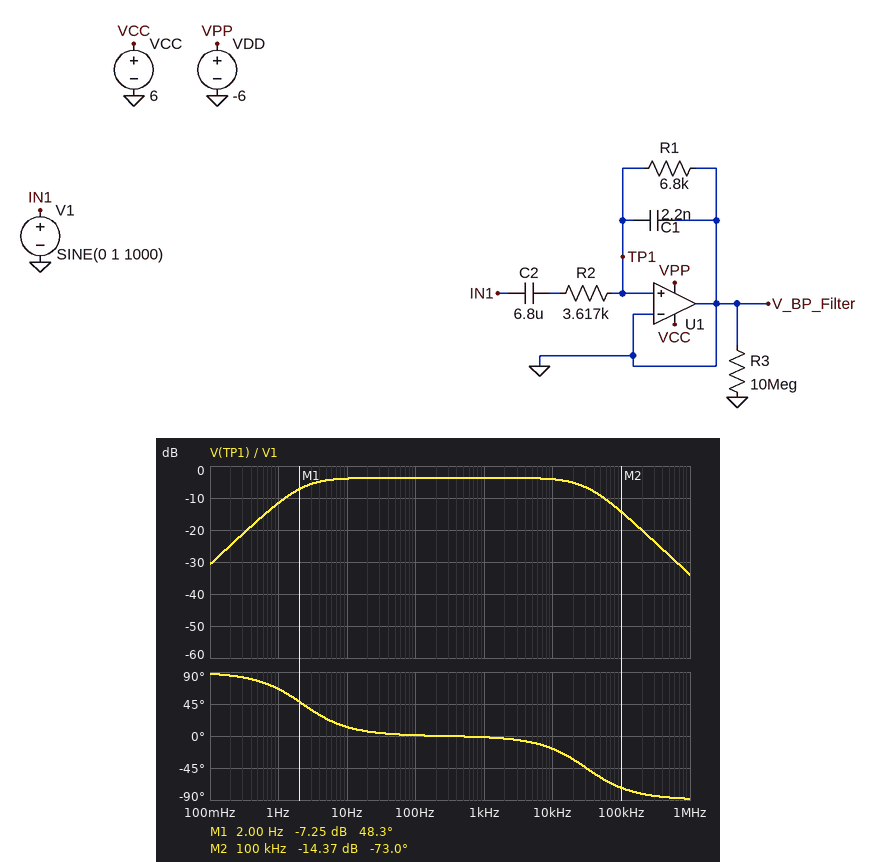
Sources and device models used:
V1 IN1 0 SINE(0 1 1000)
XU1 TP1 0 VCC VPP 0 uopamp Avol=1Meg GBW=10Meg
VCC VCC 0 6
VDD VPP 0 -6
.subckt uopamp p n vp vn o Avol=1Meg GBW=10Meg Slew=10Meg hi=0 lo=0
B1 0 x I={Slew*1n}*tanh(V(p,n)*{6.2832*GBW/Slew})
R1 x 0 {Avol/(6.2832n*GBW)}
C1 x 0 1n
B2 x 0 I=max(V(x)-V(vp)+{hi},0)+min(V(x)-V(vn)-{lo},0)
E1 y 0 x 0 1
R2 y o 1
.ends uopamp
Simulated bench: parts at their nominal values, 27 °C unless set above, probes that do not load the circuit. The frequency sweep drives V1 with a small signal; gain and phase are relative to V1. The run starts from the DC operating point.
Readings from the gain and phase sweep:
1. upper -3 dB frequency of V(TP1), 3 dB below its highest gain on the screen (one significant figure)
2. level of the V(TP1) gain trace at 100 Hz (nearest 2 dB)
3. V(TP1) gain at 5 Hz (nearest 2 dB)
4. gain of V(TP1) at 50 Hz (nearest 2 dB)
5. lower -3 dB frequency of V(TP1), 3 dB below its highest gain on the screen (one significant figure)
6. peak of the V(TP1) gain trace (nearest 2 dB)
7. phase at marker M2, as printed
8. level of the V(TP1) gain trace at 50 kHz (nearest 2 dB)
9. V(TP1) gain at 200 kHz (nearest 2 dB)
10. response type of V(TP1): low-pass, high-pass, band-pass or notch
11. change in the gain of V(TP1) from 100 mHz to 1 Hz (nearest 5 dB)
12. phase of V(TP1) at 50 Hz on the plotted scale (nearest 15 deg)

30 kHz
-4 dB
-4 dB
-4 dB
2 Hz
-4 dB
-73.0 deg
-10 dB
-20 dB
band-pass
20 dB
0 deg
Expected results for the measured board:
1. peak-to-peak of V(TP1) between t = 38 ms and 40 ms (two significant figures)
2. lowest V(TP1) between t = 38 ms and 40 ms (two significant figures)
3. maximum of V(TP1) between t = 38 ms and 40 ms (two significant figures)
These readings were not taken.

1.3 V
-650 mV
650 mV
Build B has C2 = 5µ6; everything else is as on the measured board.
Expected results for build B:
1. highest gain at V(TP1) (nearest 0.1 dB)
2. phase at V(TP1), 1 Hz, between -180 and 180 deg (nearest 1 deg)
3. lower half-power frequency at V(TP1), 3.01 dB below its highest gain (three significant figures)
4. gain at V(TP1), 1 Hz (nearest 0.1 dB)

-3.7 dB
70 deg
2.73 Hz
-13.0 dB
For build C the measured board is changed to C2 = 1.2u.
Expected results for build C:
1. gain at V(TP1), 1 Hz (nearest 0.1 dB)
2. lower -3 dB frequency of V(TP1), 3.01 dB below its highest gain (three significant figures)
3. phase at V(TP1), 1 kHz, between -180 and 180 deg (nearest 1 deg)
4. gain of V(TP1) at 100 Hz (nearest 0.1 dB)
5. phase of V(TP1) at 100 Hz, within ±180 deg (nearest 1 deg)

-25.8 dB
12.7 Hz
-1 deg
-3.8 dB
7 deg
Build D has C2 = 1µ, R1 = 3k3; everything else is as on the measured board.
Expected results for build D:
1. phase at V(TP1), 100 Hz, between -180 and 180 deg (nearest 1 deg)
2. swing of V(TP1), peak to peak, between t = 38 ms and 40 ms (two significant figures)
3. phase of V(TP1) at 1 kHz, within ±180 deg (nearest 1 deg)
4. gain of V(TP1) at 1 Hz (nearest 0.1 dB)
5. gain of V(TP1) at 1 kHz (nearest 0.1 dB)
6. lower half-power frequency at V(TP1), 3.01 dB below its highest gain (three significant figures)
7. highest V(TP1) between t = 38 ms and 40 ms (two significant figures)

13 deg
950 mV
0 deg
-33.7 dB
-6.4 dB
23.0 Hz
480 mV
